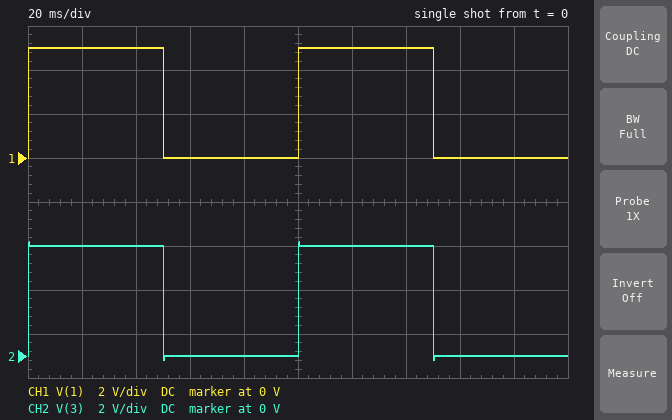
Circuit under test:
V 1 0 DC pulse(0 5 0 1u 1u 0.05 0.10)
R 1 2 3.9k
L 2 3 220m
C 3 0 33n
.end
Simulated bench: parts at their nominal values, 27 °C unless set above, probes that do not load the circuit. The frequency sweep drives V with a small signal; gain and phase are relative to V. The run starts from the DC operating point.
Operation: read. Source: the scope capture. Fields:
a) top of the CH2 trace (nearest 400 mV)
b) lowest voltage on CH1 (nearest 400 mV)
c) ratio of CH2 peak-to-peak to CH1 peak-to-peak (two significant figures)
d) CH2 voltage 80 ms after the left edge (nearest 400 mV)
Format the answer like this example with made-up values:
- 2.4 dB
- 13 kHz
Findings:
- 5.2 V
- 0 V
- 1.1
- 0 V
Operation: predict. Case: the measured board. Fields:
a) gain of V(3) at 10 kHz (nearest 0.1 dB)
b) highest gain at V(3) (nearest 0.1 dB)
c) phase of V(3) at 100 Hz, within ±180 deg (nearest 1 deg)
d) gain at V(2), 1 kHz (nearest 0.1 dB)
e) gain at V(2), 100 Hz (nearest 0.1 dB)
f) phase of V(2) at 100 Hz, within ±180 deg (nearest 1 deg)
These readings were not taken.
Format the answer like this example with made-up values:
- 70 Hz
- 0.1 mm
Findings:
- -29.2 dB
- 0 dB
- -5 deg
- -3.6 dB
- 0 dB
- -5 deg
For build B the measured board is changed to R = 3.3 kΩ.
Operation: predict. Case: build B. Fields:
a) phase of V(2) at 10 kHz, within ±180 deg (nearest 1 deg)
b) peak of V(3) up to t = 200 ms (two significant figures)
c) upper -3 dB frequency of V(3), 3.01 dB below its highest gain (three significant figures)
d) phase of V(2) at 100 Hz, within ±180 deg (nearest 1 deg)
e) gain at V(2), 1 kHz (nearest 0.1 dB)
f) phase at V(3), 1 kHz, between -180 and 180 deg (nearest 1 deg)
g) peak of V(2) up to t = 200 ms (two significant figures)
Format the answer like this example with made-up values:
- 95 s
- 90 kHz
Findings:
- 14 deg
- 5.4 V
- 2.02 kHz
- -4 deg
- -2.8 dB
- -44 deg
- 5.3 V
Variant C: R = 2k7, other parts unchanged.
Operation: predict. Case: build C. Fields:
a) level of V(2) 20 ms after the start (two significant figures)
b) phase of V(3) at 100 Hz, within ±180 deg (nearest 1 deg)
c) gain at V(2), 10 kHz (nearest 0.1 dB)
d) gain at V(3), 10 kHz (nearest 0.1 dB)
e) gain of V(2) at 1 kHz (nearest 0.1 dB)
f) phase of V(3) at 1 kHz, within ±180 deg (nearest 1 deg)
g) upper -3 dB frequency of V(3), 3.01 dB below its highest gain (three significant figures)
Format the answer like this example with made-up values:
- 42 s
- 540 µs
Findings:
- 5.0 V
- -3 deg
- -0.2 dB
- -29.0 dB
- -2.1 dB
- -38 deg
- 2.17 kHz
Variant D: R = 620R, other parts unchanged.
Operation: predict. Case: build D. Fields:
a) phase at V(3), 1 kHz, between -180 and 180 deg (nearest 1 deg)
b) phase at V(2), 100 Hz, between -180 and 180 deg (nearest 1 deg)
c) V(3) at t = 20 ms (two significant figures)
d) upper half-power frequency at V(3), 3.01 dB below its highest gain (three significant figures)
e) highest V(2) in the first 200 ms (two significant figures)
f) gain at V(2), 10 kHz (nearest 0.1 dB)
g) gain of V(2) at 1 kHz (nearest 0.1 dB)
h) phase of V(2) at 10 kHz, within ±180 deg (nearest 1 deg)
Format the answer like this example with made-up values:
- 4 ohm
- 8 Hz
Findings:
- -10 deg
- -1 deg
- 5.0 V
- 2.05 kHz
- 5.7 V
- 0 dB
- -0.1 dB
- 3 deg
